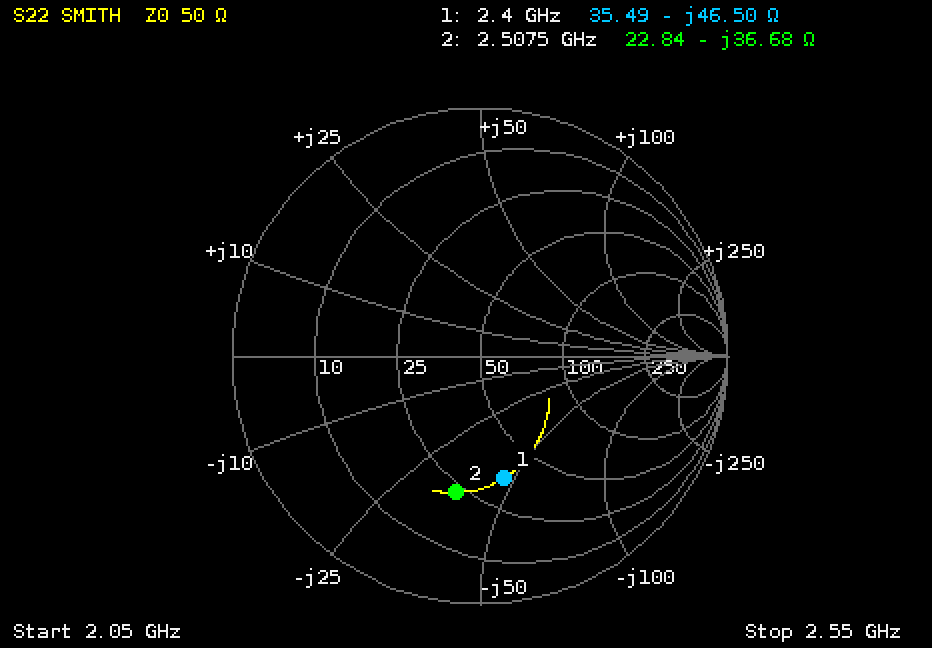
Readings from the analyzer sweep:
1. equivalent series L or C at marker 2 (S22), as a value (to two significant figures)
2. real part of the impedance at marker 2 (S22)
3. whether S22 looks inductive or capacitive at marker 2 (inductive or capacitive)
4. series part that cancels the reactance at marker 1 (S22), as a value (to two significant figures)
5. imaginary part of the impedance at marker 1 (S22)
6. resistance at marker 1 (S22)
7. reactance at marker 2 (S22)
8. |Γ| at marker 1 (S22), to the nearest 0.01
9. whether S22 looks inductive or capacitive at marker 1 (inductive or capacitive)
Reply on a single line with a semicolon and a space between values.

1.7 pF; 22.84 Ω; capacitive; 3.1 nH; -46.50 Ω; 35.49 Ω; -36.68 Ω; 0.50; capacitive
